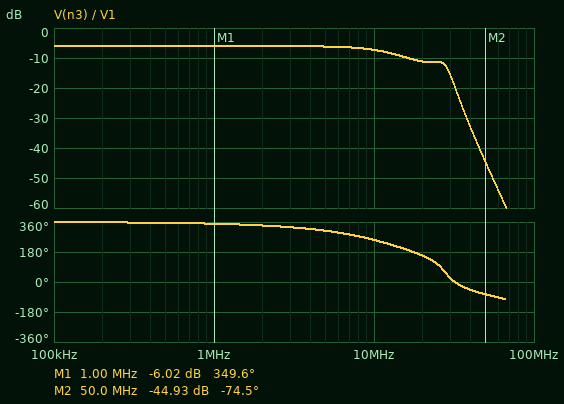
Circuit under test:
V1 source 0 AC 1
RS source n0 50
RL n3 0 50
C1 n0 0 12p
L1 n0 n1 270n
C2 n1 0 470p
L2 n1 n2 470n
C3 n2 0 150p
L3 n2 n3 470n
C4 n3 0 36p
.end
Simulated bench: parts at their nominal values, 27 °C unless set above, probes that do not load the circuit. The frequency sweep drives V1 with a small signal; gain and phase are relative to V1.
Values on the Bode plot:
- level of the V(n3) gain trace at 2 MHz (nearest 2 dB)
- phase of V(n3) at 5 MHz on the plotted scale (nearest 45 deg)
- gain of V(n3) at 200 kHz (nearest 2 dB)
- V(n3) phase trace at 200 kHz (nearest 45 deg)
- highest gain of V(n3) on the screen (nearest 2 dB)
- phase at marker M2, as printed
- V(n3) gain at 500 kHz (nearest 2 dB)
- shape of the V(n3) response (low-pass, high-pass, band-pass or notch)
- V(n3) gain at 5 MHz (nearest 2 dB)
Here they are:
-6 dB
315 deg
-6 dB
360 deg
-6 dB
-74.5 deg
-6 dB
low-pass
-6 dB
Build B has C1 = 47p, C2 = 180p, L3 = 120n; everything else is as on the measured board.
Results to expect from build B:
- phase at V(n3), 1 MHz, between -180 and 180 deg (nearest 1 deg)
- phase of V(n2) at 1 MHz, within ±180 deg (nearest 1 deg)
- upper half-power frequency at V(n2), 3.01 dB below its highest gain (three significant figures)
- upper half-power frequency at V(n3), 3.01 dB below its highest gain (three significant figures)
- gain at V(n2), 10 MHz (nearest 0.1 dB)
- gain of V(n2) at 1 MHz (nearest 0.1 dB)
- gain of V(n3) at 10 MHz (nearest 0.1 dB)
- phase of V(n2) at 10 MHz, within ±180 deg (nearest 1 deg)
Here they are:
-7 deg
-6 deg
30.5 MHz
31.2 MHz
-6.1 dB
-6.0 dB
-6.0 dB
-60 deg
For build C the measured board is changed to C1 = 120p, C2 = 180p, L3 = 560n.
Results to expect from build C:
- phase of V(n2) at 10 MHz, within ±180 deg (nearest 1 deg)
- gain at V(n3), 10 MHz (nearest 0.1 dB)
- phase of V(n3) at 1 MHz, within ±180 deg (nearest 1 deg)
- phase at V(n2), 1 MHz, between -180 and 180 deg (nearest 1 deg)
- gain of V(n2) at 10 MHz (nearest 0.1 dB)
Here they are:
-55 deg
-6.5 dB
-9 deg
-5 deg
-5.2 dB
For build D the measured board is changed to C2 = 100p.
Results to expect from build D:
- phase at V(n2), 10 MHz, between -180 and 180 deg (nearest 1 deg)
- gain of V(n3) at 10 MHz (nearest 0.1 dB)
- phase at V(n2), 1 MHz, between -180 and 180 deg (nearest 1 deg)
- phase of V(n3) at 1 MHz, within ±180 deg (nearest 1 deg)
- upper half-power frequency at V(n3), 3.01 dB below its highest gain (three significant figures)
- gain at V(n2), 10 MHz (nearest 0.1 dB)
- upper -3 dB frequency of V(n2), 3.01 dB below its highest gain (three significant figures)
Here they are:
-37 deg
-6.2 dB
-4 deg
-7 deg
35.4 MHz
-5.3 dB
40.3 MHz
